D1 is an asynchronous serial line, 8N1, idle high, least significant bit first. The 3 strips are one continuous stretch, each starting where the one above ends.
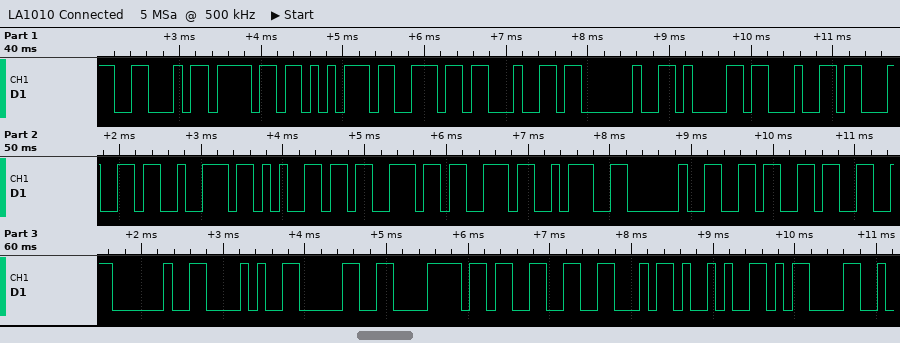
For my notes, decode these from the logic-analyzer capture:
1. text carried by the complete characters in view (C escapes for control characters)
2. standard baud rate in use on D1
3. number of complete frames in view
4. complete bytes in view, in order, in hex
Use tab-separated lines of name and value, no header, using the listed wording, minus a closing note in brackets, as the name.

text carried by the complete characters in view	"Found address: 63 (0x3F)\r"
standard baud rate in use on D1	9600 baud
number of complete frames in view	25
complete bytes in view, in order, in hex	0x46 0x6F 0x75 0x6E 0x64 0x20 0x61 0x64 0x64 0x72 0x65 0x73 0x73 0x3A 0x20 0x36 0x33 0x20 0x28 0x30 0x78 0x33 0x46 0x29 0x0D
